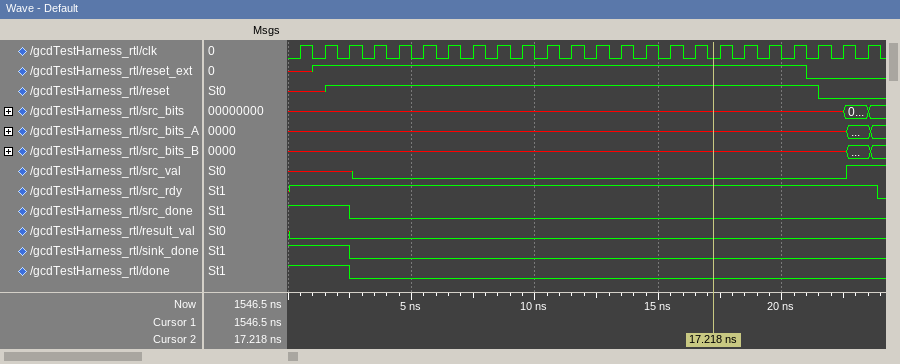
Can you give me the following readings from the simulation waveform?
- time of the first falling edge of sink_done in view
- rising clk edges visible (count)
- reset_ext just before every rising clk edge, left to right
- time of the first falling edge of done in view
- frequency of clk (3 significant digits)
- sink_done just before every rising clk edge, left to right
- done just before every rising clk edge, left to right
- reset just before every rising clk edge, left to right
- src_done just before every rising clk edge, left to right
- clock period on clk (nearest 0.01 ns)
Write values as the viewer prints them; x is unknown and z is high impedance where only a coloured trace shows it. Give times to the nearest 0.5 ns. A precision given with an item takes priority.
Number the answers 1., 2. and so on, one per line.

1. 2.5 ns
2. 24
3. x 1 1 1 1 1 1 1 1 1 1 1 1 1 1 1 1 1 1 1 1 0 0 0
4. 2.5 ns
5. 1.00 GHz
6. 1 1 1 0 0 0 0 0 0 0 0 0 0 0 0 0 0 0 0 0 0 0 0 0
7. 1 1 1 0 0 0 0 0 0 0 0 0 0 0 0 0 0 0 0 0 0 0 0 0
8. x x 1 1 1 1 1 1 1 1 1 1 1 1 1 1 1 1 1 1 1 1 0 0
9. 1 1 1 0 0 0 0 0 0 0 0 0 0 0 0 0 0 0 0 0 0 0 0 0
10. 1 ns
